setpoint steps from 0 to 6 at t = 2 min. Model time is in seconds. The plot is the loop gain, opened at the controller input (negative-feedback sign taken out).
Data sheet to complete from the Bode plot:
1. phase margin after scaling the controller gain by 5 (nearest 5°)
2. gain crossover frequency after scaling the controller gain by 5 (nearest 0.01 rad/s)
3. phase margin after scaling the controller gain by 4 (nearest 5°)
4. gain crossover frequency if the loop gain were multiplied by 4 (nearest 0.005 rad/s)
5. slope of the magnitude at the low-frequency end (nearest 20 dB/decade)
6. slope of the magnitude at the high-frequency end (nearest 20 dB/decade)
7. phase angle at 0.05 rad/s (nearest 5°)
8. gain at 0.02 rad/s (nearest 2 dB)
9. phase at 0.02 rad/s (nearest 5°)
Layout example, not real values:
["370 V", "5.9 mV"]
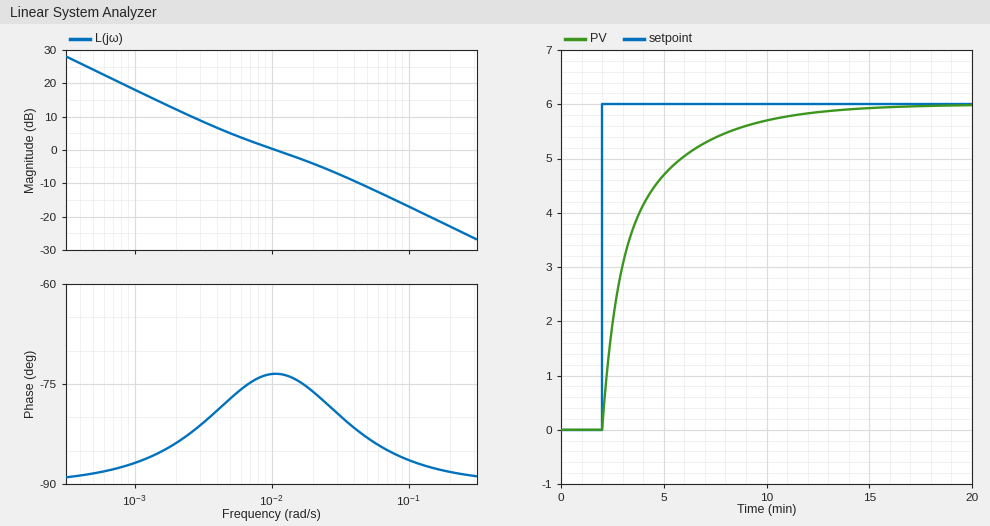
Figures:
["95°", "0.07 rad/s", "95°", "0.055 rad/s", "-20 dB/decade", "-20 dB/decade", "-85°", "-4 dB", "-75°"]
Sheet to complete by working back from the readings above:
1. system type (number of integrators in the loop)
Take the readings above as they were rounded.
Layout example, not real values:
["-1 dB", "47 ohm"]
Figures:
["1"]
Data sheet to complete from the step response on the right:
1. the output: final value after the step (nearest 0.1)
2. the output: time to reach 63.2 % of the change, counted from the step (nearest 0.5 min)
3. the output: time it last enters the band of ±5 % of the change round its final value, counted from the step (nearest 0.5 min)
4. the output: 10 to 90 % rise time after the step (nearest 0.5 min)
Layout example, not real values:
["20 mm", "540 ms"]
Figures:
["6.0", "1.5 min", "8.0 min", "5.5 min"]
